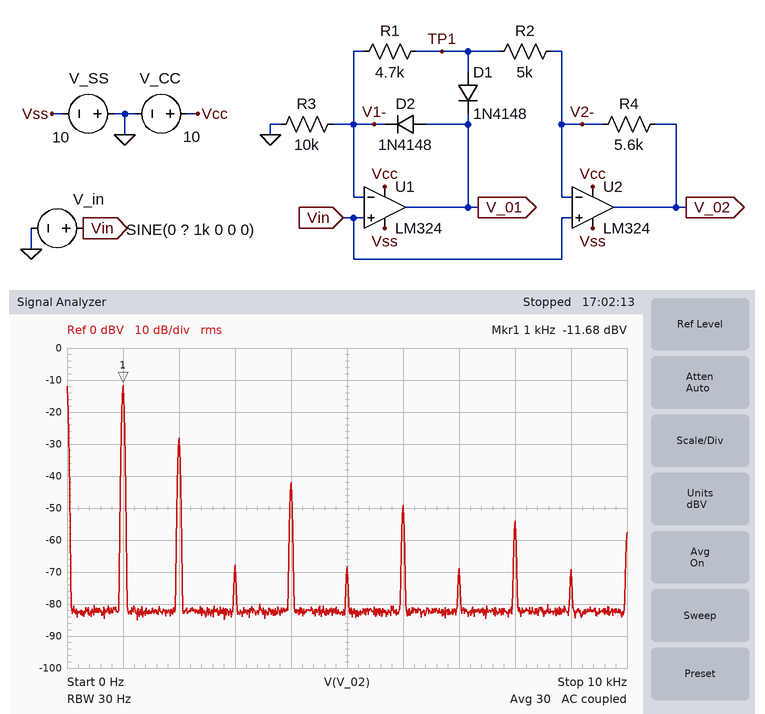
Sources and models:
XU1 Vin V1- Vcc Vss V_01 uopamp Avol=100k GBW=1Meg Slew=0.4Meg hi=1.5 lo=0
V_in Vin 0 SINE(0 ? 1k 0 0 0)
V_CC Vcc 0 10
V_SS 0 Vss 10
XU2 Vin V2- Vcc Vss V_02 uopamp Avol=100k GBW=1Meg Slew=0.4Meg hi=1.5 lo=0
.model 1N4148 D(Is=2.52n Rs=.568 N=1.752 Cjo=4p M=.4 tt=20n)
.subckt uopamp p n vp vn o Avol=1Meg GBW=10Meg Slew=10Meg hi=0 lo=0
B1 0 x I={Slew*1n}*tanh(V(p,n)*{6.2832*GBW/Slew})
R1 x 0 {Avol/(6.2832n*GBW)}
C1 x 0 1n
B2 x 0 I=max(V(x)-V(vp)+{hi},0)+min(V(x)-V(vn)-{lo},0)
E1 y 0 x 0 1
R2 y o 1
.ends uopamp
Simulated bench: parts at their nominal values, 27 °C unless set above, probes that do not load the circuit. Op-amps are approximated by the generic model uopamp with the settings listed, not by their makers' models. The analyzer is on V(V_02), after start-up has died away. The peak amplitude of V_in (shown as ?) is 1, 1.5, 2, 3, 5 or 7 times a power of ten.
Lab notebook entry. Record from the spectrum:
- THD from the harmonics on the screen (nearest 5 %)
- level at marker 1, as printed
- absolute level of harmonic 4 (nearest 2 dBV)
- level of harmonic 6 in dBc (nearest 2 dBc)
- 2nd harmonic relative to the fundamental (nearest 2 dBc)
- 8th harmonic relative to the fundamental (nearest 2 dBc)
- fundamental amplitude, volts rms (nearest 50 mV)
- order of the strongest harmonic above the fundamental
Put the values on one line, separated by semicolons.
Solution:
15 %; -11.68 dBV; -42 dBV; -38 dBc; -16 dBc; -42 dBc; 250 mV; 2
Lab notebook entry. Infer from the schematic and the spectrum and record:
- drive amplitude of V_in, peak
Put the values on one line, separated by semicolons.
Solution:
500 mV
